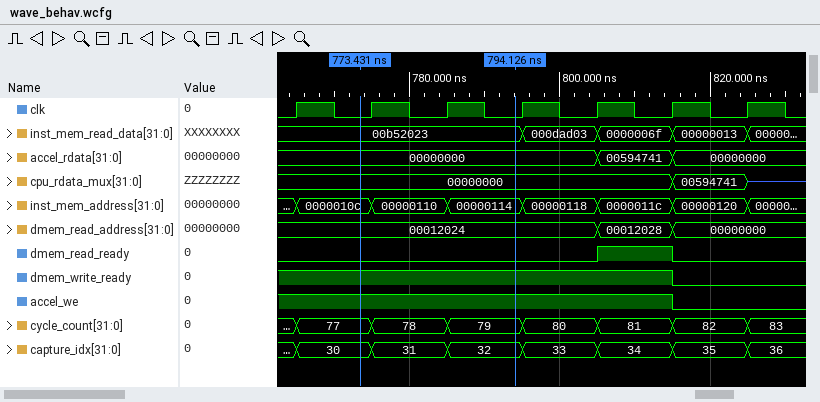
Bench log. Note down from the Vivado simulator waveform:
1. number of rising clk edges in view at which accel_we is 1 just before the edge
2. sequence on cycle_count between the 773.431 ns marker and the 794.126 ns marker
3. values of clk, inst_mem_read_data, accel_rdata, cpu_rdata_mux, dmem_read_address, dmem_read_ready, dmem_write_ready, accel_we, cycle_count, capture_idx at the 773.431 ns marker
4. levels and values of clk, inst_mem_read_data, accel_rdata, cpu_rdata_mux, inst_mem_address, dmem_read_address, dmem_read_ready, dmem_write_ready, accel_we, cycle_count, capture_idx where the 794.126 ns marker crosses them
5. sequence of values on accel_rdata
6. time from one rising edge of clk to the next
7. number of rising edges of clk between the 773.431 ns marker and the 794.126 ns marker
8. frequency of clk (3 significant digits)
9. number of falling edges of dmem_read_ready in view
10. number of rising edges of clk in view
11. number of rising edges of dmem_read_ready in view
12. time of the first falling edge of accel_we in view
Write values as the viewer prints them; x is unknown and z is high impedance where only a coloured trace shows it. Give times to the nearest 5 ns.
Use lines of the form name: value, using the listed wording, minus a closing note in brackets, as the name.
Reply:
number of rising clk edges in view at which accel_we is 1 just before the edge: 6
sequence on cycle_count between the 773.431 ns marker and the 794.126 ns marker: 77, 78, 79
values of clk, inst_mem_read_data, accel_rdata, cpu_rdata_mux, dmem_read_address, dmem_read_ready, dmem_write_ready, accel_we, cycle_count, capture_idx at the 773.431 ns marker: clk=0, inst_mem_read_data=00b52023, accel_rdata=00000000, cpu_rdata_mux=00000000, dmem_read_address=00012024, dmem_read_ready=0, dmem_write_ready=1, accel_we=1, cycle_count=77, capture_idx=30
levels and values of clk, inst_mem_read_data, accel_rdata, cpu_rdata_mux, inst_mem_address, dmem_read_address, dmem_read_ready, dmem_write_ready, accel_we, cycle_count, capture_idx where the 794.126 ns marker crosses them: clk=0, inst_mem_read_data=00b52023, accel_rdata=00000000, cpu_rdata_mux=00000000, inst_mem_address=00000114, dmem_read_address=00012024, dmem_read_ready=0, dmem_write_ready=1, accel_we=1, cycle_count=79, capture_idx=32
sequence of values on accel_rdata: 00000000, 00594741, 00000000
time from one rising edge of clk to the next: 10 ns
number of rising edges of clk between the 773.431 ns marker and the 794.126 ns marker: 2
frequency of clk: 100 MHz
number of falling edges of dmem_read_ready in view: 1
number of rising edges of clk in view: 7
number of rising edges of dmem_read_ready in view: 1
time of the first falling edge of accel_we in view: 815 ns
